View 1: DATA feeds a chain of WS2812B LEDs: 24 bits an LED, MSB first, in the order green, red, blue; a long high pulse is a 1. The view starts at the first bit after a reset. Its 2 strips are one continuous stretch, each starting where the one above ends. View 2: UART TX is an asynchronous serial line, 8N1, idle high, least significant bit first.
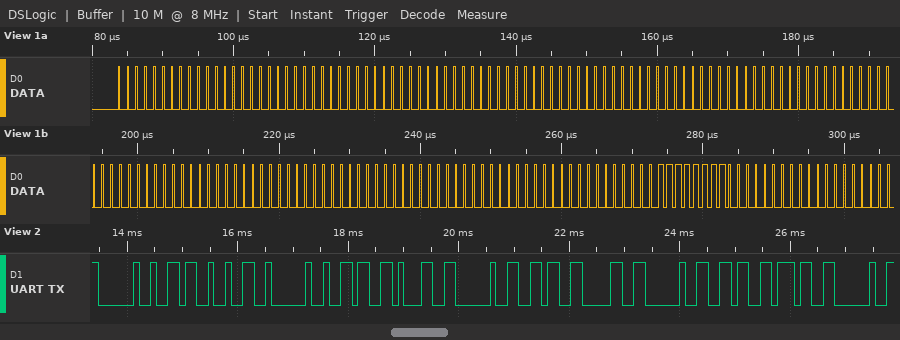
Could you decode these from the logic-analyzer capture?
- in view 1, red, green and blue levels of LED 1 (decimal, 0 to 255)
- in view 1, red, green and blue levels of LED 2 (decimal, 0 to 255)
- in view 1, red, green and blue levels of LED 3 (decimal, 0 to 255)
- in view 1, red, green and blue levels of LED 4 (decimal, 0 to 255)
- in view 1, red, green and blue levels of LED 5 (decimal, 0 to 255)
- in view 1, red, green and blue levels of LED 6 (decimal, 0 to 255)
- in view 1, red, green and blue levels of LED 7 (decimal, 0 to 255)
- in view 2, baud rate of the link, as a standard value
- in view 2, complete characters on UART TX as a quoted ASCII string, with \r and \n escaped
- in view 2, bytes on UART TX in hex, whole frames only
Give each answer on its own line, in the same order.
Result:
0, 0, 0
0, 0, 0
0, 0, 0
0, 0, 0
0, 0, 0
0, 0, 0
255, 0, 0
9600 baud
" 62 61 60 67 "
20 36 32 20 36 31 20 36 30 20 36 37 20
